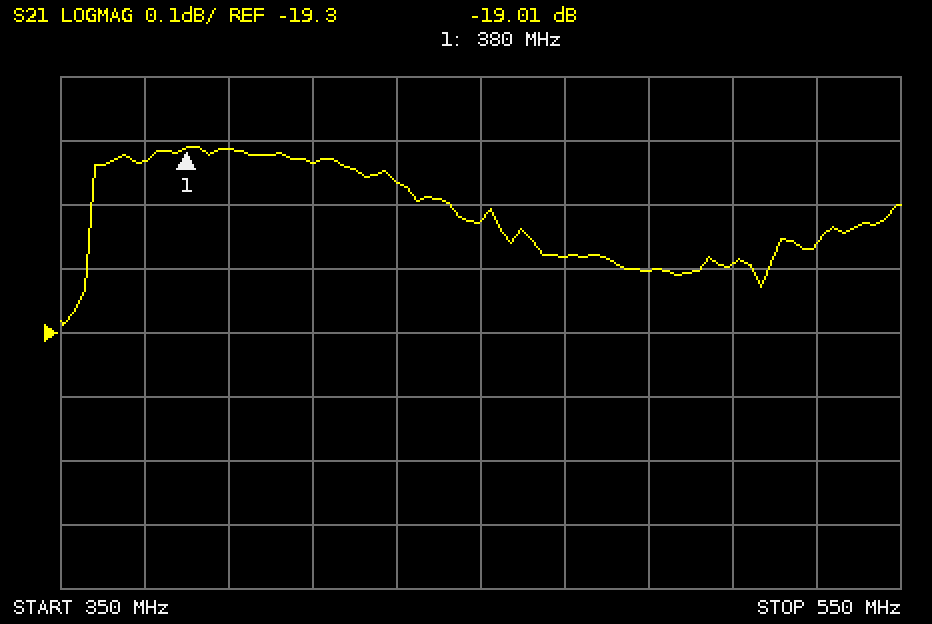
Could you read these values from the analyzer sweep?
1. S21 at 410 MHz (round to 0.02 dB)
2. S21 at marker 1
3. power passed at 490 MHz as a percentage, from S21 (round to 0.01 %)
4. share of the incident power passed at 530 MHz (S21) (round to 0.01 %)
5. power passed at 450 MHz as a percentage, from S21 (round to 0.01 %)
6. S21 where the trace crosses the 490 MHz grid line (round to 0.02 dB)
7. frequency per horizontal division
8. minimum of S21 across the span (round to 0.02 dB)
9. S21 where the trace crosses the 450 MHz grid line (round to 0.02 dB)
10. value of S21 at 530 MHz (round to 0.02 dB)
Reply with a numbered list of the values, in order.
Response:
1. -19.04 dB
2. -19.01 dB
3. 1.20 %
4. 1.21 %
5. 1.22 %
6. -19.20 dB
7. 20 MHz
8. -19.28 dB
9. -19.12 dB
10. -19.16 dB
